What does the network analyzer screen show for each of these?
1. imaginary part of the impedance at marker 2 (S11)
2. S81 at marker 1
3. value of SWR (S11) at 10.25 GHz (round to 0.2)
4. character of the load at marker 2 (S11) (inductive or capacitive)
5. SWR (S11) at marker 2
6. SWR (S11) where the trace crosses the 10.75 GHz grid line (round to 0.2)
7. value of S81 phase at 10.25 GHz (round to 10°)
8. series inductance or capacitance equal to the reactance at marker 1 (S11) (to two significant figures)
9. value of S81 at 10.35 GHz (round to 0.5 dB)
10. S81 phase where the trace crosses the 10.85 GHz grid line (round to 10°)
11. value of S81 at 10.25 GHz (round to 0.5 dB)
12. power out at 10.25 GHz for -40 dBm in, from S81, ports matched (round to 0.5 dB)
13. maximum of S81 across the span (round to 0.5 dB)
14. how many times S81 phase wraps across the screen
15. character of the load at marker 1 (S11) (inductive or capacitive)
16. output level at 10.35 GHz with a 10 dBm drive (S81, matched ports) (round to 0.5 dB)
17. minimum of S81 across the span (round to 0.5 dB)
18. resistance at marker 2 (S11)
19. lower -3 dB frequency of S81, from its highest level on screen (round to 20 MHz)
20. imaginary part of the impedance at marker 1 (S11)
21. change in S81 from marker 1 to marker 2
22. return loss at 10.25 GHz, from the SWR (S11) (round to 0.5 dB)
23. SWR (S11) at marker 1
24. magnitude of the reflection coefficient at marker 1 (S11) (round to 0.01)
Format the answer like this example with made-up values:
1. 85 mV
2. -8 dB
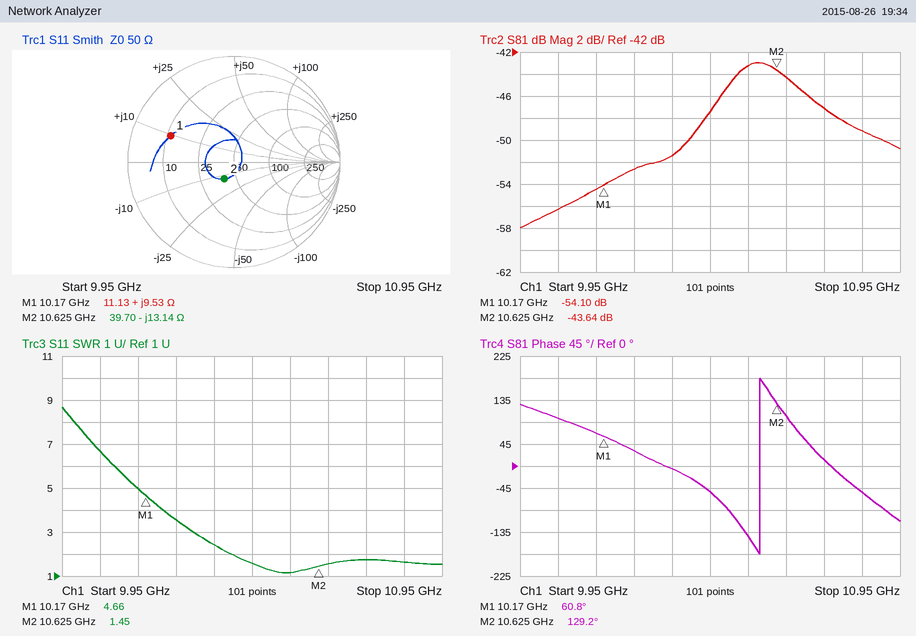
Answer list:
1. -13.14 Ω
2. -54.10 dB
3. 3.6
4. capacitive
5. 1.45
6. 1.8
7. 30°
8. 150 pH
9. -51.5 dB
10. -50°
11. -52.5 dB
12. -92.5 dBm
13. -43.0 dB
14. 1
15. inductive
16. -41.5 dBm
17. -58.0 dB
18. 39.70 Ω
19. 10.48 GHz
20. +9.53 Ω
21. 10.46 dB
22. 5.0 dB
23. 4.66
24. 0.65
